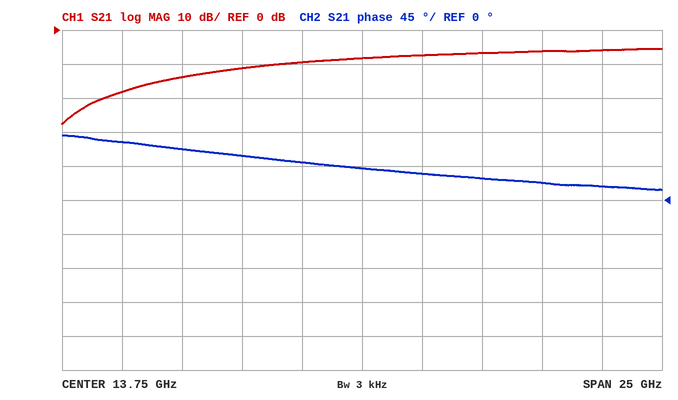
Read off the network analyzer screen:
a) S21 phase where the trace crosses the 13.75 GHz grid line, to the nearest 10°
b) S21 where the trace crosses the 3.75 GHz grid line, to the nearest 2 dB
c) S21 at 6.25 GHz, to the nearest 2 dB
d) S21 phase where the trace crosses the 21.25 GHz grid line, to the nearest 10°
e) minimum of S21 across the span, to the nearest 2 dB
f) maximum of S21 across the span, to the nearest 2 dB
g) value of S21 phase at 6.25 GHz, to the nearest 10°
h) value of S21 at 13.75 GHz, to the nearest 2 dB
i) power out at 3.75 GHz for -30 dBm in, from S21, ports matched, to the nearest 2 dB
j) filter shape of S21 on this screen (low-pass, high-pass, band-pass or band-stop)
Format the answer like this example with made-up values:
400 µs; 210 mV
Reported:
40°; -18 dB; -14 dB; 20°; -28 dB; -6 dB; 70°; -8 dB; -48 dBm; high-pass
